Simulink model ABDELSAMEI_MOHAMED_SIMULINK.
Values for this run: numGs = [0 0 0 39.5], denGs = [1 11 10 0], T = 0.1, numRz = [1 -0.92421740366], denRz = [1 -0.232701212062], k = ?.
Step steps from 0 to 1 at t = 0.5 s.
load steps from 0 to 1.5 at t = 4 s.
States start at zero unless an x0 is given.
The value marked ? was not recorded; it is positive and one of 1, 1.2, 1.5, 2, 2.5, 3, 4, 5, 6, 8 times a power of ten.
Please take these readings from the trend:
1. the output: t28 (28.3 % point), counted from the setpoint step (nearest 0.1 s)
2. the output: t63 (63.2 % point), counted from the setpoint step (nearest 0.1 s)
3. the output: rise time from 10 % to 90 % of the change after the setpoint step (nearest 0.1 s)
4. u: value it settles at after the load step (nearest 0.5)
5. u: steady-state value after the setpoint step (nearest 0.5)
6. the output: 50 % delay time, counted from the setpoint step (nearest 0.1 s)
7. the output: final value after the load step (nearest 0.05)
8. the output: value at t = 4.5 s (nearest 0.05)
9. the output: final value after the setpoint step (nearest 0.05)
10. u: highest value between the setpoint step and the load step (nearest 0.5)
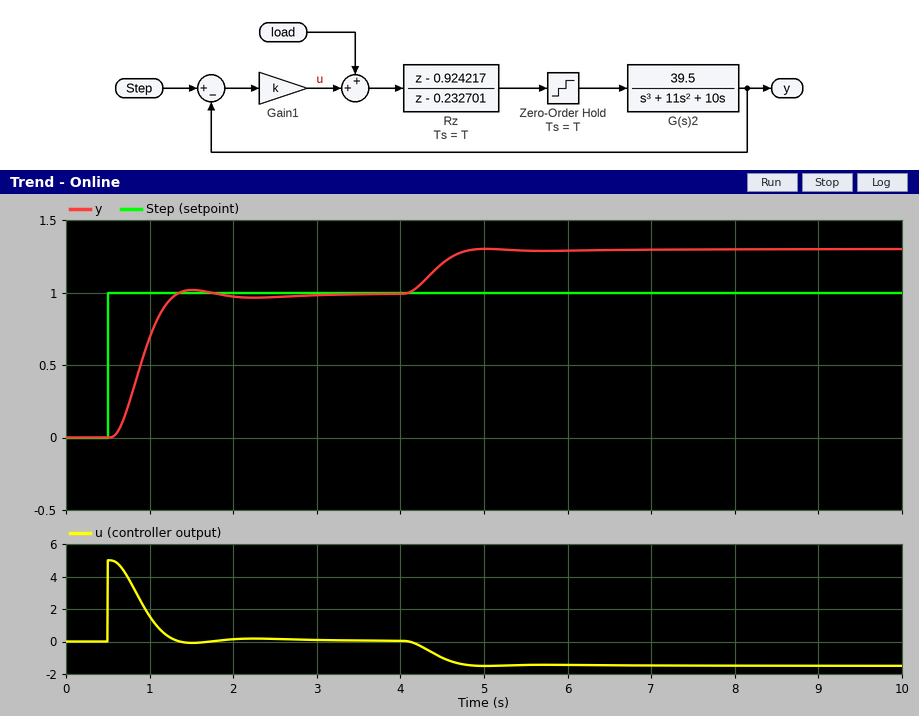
0.3 s
0.5 s
0.5 s
-1.5
0.0
0.4 s
1.30
1.20
1.00
5.0
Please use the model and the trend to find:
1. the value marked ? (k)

5
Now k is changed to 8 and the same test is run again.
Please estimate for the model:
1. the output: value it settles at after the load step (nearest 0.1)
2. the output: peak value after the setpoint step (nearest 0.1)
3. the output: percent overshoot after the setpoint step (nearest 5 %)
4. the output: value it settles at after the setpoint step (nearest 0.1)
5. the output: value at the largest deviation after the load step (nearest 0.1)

1.2
1.2
20 %
1.0
1.2
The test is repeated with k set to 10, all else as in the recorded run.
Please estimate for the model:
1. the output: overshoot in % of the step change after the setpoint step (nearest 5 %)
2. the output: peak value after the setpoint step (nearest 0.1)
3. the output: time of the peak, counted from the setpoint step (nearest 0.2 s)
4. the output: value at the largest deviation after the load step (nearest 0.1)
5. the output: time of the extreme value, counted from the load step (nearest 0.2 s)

35 %
1.3
0.6 s
1.2
0.6 s
